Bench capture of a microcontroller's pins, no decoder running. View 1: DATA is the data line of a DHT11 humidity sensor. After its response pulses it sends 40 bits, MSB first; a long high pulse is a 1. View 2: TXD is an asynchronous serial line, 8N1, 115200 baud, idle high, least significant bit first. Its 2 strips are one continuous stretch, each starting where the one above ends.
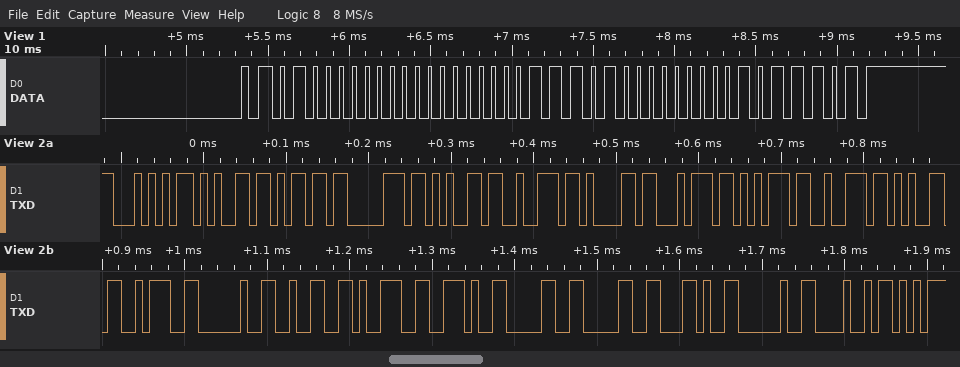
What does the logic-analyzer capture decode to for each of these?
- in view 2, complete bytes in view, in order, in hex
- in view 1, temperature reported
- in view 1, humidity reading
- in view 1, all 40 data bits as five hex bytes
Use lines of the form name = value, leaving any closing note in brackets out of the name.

in view 2, complete bytes in view, in order, in hex = 54 65 6D 70 65 72 61 74 75 72 65 3A 20 32 39 2E 30 30 2C 20 48
in view 1, temperature reported = 29.0 °C
in view 1, humidity reading = 64 %
in view 1, all 40 data bits as five hex bytes = 40 00 1D 00 5D
